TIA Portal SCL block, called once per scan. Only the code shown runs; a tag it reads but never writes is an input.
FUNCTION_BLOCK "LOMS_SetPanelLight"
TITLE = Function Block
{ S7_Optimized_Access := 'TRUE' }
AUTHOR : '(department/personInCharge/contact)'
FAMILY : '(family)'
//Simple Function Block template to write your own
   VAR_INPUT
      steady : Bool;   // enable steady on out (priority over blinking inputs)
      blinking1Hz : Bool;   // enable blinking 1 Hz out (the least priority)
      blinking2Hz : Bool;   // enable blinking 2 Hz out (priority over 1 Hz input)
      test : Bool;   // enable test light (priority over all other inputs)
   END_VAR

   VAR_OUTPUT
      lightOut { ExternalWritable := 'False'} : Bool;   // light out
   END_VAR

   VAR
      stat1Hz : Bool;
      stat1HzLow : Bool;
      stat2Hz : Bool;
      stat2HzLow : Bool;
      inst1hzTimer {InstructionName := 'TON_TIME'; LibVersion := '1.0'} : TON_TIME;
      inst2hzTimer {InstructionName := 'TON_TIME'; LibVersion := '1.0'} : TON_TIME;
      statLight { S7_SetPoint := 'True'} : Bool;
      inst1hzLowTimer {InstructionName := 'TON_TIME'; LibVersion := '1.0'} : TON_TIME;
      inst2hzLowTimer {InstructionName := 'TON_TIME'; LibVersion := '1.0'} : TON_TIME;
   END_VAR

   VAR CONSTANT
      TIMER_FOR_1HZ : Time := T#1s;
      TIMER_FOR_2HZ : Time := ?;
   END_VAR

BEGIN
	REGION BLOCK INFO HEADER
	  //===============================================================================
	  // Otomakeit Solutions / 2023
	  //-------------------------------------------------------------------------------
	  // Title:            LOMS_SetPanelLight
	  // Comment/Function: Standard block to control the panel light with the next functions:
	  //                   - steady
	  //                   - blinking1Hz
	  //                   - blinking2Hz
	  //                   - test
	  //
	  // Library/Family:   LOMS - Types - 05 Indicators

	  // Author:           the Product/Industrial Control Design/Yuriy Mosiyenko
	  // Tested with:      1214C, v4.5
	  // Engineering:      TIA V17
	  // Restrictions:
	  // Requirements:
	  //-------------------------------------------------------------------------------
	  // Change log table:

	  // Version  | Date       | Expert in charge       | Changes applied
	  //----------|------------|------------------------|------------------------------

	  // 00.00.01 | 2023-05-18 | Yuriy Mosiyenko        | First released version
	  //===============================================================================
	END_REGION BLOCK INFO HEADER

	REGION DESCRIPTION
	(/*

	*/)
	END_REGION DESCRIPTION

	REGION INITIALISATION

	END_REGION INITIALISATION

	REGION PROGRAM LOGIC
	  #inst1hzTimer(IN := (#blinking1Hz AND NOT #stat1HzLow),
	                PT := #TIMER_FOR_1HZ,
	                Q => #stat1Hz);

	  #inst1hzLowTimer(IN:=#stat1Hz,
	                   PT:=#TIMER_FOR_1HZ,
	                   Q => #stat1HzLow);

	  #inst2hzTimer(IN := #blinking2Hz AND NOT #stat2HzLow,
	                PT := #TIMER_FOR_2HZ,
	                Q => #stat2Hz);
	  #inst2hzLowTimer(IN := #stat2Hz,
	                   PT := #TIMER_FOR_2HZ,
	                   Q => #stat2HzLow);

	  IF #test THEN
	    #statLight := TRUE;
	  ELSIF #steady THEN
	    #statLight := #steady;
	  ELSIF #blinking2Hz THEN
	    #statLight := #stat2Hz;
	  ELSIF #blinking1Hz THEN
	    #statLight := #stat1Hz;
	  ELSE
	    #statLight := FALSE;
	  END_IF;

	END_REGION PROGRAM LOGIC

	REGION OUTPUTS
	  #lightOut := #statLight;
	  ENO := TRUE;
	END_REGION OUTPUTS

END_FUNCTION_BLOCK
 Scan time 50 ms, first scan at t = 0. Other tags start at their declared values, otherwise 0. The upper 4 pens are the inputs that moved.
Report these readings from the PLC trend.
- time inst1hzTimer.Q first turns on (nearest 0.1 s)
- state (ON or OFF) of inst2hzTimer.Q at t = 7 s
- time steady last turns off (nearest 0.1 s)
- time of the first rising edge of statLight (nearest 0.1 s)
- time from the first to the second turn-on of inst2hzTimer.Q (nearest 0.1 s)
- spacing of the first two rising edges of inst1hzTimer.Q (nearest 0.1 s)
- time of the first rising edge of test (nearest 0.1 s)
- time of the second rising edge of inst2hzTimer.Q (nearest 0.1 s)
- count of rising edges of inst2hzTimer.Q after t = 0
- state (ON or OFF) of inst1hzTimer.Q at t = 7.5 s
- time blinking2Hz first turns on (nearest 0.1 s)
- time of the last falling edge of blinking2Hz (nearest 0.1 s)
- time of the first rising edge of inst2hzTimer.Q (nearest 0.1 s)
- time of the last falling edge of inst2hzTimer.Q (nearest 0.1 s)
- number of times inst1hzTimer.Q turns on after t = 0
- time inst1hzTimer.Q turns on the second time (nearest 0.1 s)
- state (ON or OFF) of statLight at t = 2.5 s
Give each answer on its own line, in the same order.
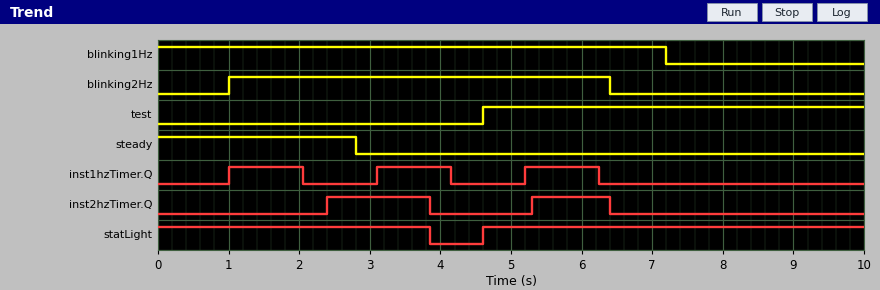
1.0 s
OFF
2.8 s
4.6 s
2.9 s
2.1 s
4.6 s
5.3 s
2
OFF
1.0 s
6.4 s
2.4 s
6.4 s
3
3.1 s
ON
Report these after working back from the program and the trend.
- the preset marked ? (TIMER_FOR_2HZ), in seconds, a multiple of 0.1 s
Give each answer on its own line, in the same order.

1.4 s
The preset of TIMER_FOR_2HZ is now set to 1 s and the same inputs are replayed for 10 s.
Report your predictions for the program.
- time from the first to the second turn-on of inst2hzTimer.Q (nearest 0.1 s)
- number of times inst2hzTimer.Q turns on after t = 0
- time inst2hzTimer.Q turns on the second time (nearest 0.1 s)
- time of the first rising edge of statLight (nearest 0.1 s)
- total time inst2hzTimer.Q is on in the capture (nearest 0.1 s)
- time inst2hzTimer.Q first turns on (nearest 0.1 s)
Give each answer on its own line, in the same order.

2.1 s
3
4.1 s
4.1 s
2.3 s
2.0 s
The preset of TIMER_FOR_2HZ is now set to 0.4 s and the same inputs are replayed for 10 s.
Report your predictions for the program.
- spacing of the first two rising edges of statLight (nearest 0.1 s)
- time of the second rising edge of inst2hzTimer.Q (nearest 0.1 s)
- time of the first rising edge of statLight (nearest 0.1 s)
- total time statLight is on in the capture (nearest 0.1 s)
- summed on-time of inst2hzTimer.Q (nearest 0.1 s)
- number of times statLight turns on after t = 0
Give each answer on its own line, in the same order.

0.9 s
2.3 s
3.2 s
9.1 s
2.7 s
3
